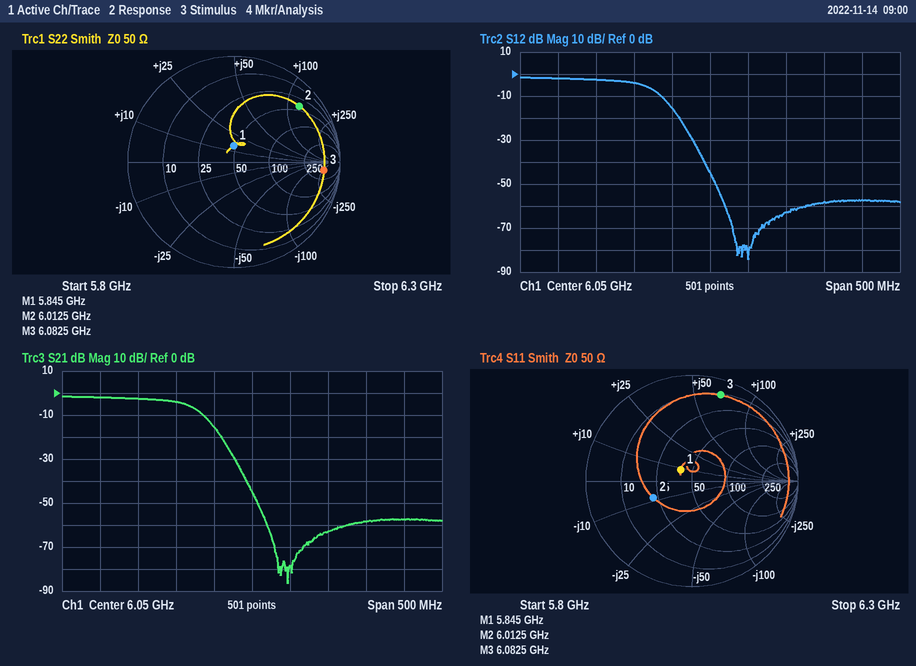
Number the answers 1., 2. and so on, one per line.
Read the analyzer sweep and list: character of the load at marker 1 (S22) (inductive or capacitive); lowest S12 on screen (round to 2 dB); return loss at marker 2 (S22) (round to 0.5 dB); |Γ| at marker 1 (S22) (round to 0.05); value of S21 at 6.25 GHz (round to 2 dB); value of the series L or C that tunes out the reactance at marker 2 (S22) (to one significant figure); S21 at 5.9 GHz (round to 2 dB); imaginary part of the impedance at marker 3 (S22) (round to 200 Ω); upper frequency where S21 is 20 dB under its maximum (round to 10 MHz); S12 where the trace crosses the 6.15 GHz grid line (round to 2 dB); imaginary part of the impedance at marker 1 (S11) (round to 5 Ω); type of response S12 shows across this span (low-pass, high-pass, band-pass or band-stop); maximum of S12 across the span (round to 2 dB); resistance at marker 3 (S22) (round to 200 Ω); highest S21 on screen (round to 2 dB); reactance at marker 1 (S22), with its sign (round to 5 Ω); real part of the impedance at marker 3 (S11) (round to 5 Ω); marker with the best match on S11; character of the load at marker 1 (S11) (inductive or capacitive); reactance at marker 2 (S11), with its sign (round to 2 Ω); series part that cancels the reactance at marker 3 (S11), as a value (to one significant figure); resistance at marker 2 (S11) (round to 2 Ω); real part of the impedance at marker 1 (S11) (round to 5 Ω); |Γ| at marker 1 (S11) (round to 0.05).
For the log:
1. inductive
2. -84 dB
3. 2.0 dB
4. 0.15
5. -58 dB
6. 200 fF
7. -2 dB
8. -200 Ω
9. 6.01 GHz
10. -62 dB
11. +10 Ω
12. low-pass
13. -2 dB
14. 400 Ω
15. -2 dB
16. +15 Ω
17. 10 Ω
18. marker 1
19. inductive
20. -8 Ω
21. 400 fF
22. 22 Ω
23. 40 Ω
24. 0.15
